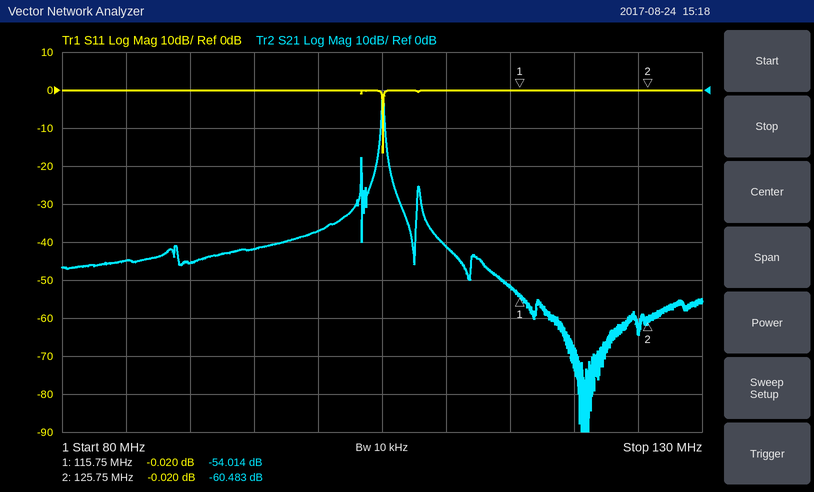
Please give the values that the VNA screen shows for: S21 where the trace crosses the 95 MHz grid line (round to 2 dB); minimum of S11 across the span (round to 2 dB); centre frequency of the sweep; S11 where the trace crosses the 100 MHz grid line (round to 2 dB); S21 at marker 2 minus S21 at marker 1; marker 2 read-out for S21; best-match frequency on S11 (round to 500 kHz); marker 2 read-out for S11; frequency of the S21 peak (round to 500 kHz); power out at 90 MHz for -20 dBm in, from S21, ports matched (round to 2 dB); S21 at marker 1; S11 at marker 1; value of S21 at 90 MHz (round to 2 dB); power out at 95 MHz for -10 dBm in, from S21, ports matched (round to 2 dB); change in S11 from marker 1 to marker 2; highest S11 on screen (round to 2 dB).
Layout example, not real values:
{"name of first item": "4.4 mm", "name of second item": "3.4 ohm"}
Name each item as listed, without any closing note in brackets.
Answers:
{"S21 where the trace crosses the 95 MHz grid line": "-42 dB", "minimum of S11 across the span": "-16 dB", "centre frequency of the sweep": "105 MHz", "S11 where the trace crosses the 100 MHz grid line": "0 dB", "S21 at marker 2 minus S21 at marker 1": "-6.469 dB", "marker 2 read-out for S21": "-60.483 dB", "best-match frequency on S11": "105.0 MHz", "marker 2 read-out for S11": "-0.020 dB", "frequency of the S21 peak": "105.0 MHz", "power out at 90 MHz for -20 dBm in, from S21, ports matched": "-66 dBm", "S21 at marker 1": "-54.014 dB", "S11 at marker 1": "-0.020 dB", "value of S21 at 90 MHz": "-46 dB", "power out at 95 MHz for -10 dBm in, from S21, ports matched": "-52 dBm", "change in S11 from marker 1 to marker 2": "0.000 dB", "highest S11 on screen": "0 dB"}
